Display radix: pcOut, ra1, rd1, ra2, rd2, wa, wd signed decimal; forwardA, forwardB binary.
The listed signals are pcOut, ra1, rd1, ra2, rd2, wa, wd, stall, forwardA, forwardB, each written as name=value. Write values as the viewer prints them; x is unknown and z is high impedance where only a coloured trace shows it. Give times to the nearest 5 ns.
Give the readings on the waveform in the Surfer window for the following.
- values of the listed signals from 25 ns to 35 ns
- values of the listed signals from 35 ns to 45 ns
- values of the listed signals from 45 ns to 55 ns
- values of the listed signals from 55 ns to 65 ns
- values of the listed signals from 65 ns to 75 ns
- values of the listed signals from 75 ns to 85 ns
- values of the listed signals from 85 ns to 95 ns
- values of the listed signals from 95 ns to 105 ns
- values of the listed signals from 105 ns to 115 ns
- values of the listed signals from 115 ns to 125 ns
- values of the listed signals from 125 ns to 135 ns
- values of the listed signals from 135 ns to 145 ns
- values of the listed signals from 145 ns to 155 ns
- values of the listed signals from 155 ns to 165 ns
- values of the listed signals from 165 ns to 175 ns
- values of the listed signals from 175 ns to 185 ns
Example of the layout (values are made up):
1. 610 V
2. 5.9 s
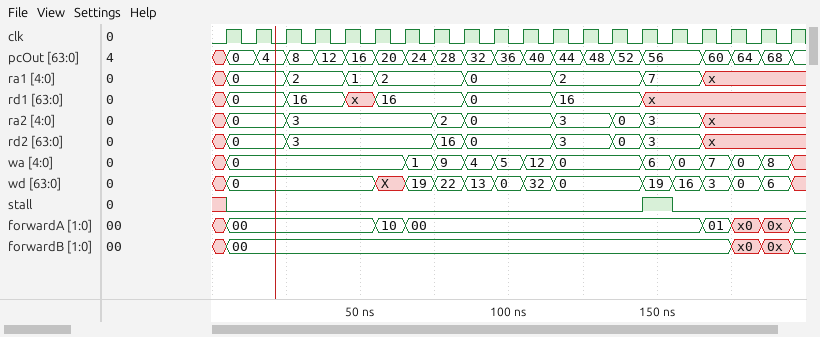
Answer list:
1. pcOut=8, ra1=2, rd1=16, ra2=3, rd2=3, wa=0, wd=0, stall=0, forwardA=00, forwardB=00
2. pcOut=12, ra1=2, rd1=16, ra2=3, rd2=3, wa=0, wd=0, stall=0, forwardA=00, forwardB=00
3. pcOut=16, ra1=1, rd1=x, ra2=3, rd2=3, wa=0, wd=0, stall=0, forwardA=00, forwardB=00
4. pcOut=20, ra1=2, rd1=16, ra2=3, rd2=3, wa=0, wd=X, stall=0, forwardA=10, forwardB=00
5. pcOut=24, ra1=2, rd1=16, ra2=3, rd2=3, wa=1, wd=19, stall=0, forwardA=00, forwardB=00
6. pcOut=28, ra1=2, rd1=16, ra2=2, rd2=16, wa=9, wd=22, stall=0, forwardA=00, forwardB=00
7. pcOut=32, ra1=0, rd1=0, ra2=0, rd2=0, wa=4, wd=13, stall=0, forwardA=00, forwardB=00
8. pcOut=36, ra1=0, rd1=0, ra2=0, rd2=0, wa=5, wd=0, stall=0, forwardA=00, forwardB=00
9. pcOut=40, ra1=0, rd1=0, ra2=0, rd2=0, wa=12, wd=32, stall=0, forwardA=00, forwardB=00
10. pcOut=44, ra1=2, rd1=16, ra2=3, rd2=3, wa=0, wd=0, stall=0, forwardA=00, forwardB=00
11. pcOut=48, ra1=2, rd1=16, ra2=3, rd2=3, wa=0, wd=0, stall=0, forwardA=00, forwardB=00
12. pcOut=52, ra1=2, rd1=16, ra2=0, rd2=0, wa=0, wd=0, stall=0, forwardA=00, forwardB=00
13. pcOut=56, ra1=7, rd1=x, ra2=3, rd2=3, wa=6, wd=19, stall=1, forwardA=00, forwardB=00
14. pcOut=56, ra1=7, rd1=x, ra2=3, rd2=3, wa=0, wd=16, stall=0, forwardA=00, forwardB=00
15. pcOut=60, ra1=x, rd1=x, ra2=x, rd2=x, wa=7, wd=3, stall=0, forwardA=01, forwardB=00
16. pcOut=64, ra1=x, rd1=x, ra2=x, rd2=x, wa=0, wd=0, stall=0, forwardA=x0, forwardB=x0
